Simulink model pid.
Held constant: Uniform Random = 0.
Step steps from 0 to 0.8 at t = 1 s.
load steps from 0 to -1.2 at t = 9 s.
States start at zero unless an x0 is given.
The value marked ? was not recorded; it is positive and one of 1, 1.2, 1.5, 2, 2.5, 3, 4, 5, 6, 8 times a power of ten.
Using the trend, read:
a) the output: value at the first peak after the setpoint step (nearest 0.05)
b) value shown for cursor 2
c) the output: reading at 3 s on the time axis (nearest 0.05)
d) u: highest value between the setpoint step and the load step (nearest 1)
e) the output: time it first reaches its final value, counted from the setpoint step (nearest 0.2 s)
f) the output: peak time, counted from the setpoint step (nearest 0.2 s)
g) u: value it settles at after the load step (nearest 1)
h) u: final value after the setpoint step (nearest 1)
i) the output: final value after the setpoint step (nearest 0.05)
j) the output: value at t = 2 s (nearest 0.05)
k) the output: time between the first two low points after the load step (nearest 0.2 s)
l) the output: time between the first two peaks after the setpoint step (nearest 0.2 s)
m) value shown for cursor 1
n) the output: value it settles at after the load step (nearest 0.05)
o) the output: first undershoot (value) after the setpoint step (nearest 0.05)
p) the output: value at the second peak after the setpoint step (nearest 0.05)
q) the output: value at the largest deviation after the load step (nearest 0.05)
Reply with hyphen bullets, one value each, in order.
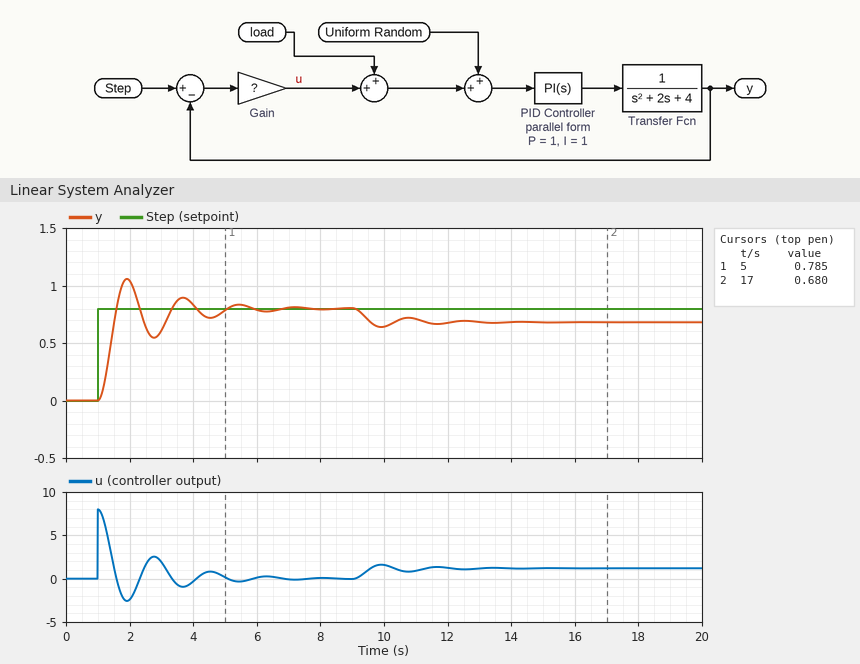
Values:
- 1.05
- 0.680
- 0.60
- 8
- 0.6 s
- 1.0 s
- 1
- 0
- 0.80
- 1.05
- 1.8 s
- 1.8 s
- 0.785
- 0.70
- 0.55
- 0.90
- 0.65
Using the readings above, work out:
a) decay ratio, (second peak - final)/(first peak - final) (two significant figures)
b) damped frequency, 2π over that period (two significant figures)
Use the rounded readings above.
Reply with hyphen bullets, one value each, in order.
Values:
- 0.40
- 3.5 rad/s
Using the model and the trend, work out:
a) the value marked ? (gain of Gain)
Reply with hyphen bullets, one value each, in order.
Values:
- 10
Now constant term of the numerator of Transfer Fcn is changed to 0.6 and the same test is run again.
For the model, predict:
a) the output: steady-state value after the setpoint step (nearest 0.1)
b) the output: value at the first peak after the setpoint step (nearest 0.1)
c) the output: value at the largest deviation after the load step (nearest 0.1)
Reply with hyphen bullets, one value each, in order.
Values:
- 0.8
- 0.9
- 0.7
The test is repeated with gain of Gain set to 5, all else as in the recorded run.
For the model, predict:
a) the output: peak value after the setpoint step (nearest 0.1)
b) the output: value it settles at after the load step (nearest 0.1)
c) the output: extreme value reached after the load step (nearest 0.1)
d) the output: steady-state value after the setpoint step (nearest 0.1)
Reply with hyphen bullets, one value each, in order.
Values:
- 0.9
- 0.6
- 0.5
- 0.8
